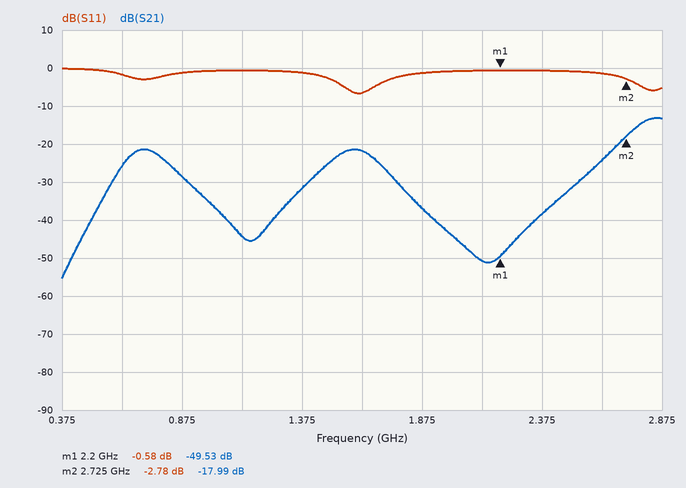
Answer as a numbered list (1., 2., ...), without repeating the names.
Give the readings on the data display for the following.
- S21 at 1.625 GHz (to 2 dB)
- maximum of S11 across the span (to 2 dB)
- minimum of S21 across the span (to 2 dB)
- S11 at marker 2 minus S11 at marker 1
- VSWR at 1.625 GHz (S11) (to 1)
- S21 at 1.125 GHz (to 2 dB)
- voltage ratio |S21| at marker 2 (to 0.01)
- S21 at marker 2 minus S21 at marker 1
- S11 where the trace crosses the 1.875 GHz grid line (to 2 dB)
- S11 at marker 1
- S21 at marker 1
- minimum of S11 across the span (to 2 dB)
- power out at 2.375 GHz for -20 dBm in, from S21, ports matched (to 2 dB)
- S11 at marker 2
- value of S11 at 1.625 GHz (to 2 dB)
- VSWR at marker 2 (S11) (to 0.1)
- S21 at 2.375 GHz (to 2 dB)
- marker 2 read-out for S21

1. -22 dB
2. 0 dB
3. -56 dB
4. -2.20 dB
5. 3
6. -44 dB
7. 0.13
8. 31.54 dB
9. -2 dB
10. -0.58 dB
11. -49.53 dB
12. -6 dB
13. -58 dBm
14. -2.78 dB
15. -6 dB
16. 6.3
17. -38 dB
18. -17.99 dB
